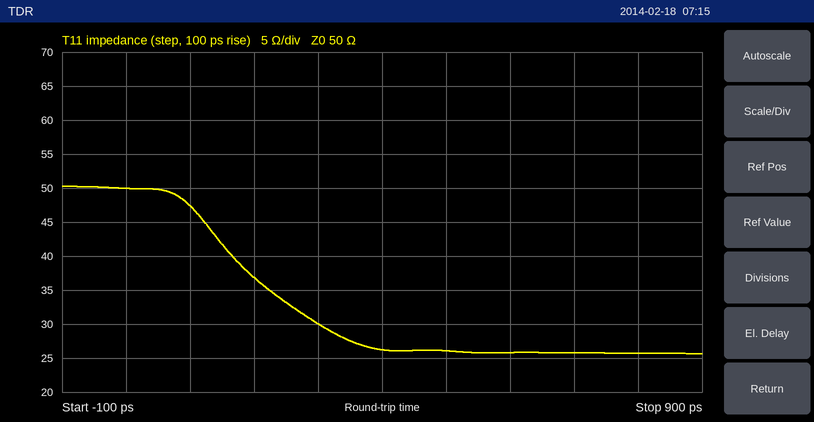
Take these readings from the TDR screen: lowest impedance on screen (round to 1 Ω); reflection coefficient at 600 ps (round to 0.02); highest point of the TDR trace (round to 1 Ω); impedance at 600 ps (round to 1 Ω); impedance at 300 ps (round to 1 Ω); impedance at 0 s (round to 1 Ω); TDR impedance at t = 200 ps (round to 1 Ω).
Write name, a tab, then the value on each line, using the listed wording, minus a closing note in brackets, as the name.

lowest impedance on screen	26 Ω
reflection coefficient at 600 ps	-0.32
highest point of the TDR trace	50 Ω
impedance at 600 ps	26 Ω
impedance at 300 ps	30 Ω
impedance at 0 s	50 Ω
TDR impedance at t = 200 ps	37 Ω
